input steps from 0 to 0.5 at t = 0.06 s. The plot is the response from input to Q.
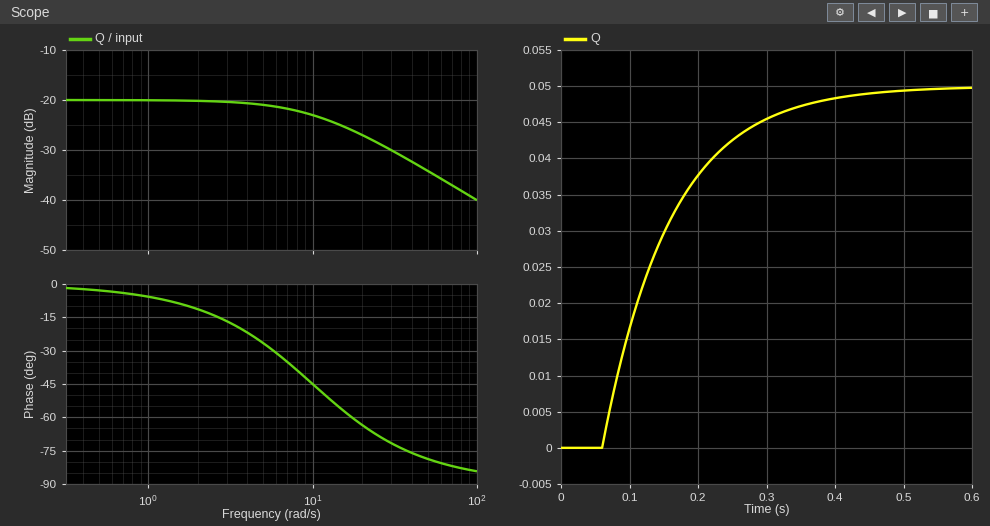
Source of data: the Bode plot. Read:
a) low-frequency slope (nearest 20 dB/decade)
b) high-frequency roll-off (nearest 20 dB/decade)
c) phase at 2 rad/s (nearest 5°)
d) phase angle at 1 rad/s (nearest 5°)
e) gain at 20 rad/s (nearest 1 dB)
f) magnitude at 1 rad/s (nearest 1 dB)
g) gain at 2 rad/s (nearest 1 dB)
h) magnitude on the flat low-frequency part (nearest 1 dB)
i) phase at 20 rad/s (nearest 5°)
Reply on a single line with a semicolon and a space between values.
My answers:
0 dB/decade; -20 dB/decade; -10°; -5°; -27 dB; -20 dB; -20 dB; -20 dB; -65°
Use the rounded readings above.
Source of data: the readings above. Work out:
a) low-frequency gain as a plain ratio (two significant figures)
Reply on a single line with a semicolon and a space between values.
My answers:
0.10
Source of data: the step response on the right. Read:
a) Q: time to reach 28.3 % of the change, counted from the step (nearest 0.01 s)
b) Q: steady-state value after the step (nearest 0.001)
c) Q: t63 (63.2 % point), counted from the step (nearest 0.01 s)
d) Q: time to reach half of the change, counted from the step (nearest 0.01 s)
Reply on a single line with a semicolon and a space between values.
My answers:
0.03 s; 0.050; 0.10 s; 0.07 s
